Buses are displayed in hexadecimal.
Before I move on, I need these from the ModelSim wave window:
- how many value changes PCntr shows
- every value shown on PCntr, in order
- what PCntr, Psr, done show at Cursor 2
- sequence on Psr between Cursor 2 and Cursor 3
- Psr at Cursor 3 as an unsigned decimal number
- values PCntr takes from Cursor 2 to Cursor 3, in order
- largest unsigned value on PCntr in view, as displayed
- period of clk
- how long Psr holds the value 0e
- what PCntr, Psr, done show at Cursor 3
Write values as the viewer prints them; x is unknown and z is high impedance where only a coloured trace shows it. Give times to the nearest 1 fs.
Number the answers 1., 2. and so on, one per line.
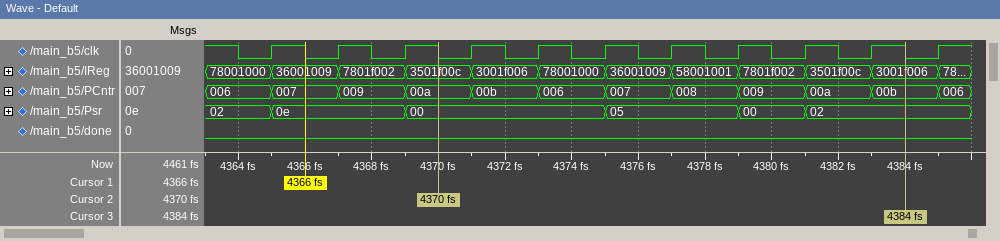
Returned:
1. 11
2. 006, 007, 009, 00a, 00b, 006, 007, 008, 009, 00a, 00b, 006
3. PCntr=00a, Psr=00, done=0
4. 00, 05, 00, 02
5. 2
6. 00a, 00b, 006, 007, 008, 009, 00a, 00b
7. 00b
8. 2 fs
9. 4 fs
10. PCntr=00b, Psr=02, done=0
